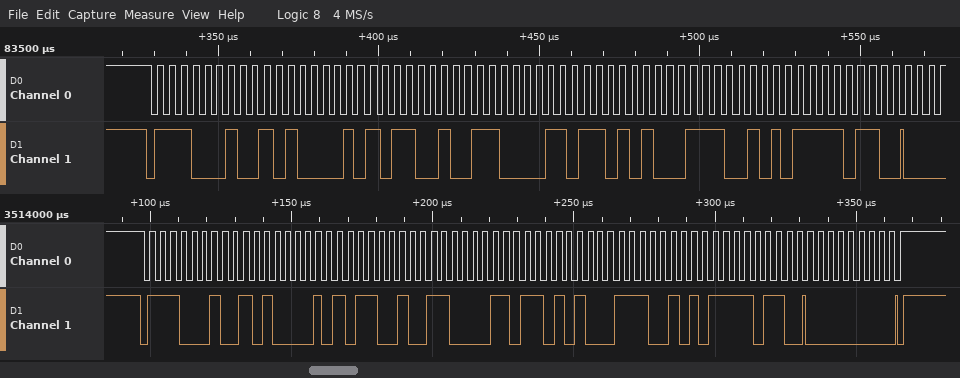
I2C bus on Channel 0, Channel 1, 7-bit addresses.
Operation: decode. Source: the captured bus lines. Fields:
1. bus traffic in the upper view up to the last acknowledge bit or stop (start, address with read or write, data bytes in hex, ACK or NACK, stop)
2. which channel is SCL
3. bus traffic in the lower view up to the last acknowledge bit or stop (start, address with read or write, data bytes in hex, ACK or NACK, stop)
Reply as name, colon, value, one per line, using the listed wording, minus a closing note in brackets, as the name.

bus traffic in the upper view up to the last acknowledge bit or stop: start, address 71 write ACK, A1 ACK, B2 ACK, C3 ACK, D4 ACK, E5 ACK, F6 ACK
which channel is SCL: Channel 0
bus traffic in the lower view up to the last acknowledge bit or stop: start, address 71 write ACK, A1 ACK, B2 ACK, C3 ACK, D4 ACK, E5 ACK, F6 ACK, 00 ACK, stop
